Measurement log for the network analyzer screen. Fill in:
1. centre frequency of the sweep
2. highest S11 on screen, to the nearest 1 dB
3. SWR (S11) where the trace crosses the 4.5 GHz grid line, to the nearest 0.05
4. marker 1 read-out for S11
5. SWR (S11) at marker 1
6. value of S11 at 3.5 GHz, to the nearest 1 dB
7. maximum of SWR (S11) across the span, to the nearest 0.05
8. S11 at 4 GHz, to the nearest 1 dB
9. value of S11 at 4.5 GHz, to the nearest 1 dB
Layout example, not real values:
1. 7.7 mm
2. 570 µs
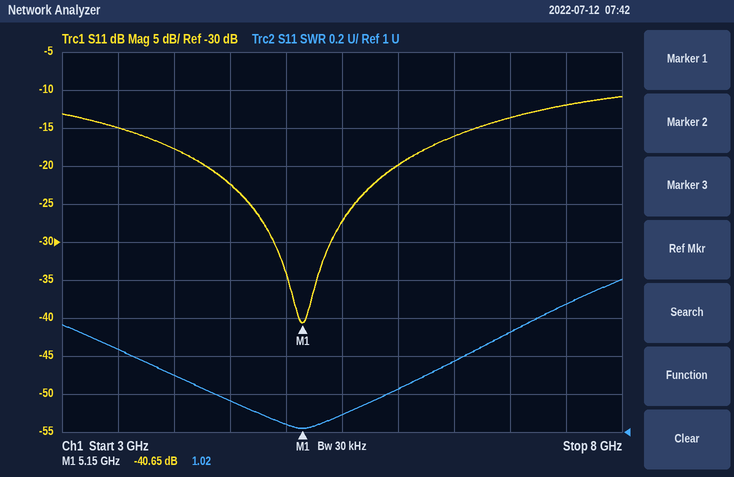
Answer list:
1. 5.5 GHz
2. -11 dB
3. 1.15
4. -40.65 dB
5. 1.02
6. -15 dB
7. 1.80
8. -18 dB
9. -22 dB
